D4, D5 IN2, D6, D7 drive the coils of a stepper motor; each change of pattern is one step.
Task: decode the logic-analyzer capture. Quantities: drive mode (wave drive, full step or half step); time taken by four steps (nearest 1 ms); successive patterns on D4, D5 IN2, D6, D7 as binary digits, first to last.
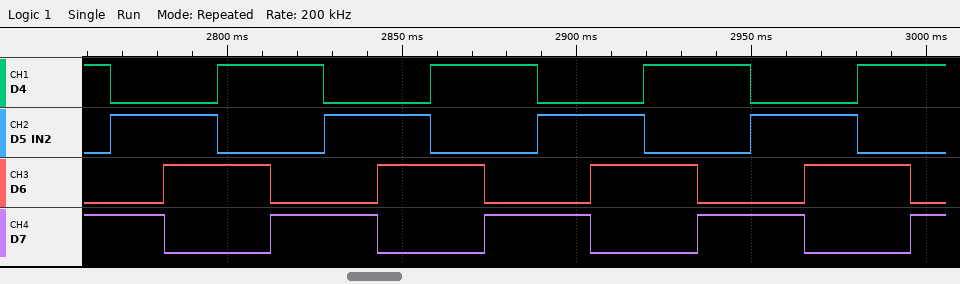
full step
61 ms
1001 0101 0110 1010 1001 0101 0110 1010 1001 0101 0110 1010 1001 0101 0110 1010 1001
